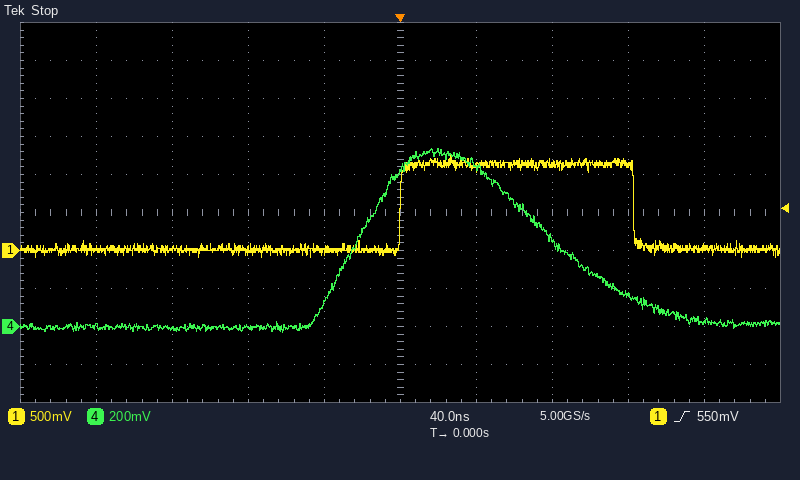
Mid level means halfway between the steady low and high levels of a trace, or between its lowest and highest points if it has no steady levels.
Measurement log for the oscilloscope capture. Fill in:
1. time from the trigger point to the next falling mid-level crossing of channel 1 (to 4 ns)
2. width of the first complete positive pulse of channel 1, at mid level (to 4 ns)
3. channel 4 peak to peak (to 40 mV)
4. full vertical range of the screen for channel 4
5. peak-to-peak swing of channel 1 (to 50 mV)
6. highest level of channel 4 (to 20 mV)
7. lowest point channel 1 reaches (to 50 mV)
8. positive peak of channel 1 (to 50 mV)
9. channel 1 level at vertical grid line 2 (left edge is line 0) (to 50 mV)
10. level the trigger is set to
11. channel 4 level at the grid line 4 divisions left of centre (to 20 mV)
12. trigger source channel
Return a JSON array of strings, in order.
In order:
["124 ns", "124 ns", "960 mV", "2 V", "1.35 V", "940 mV", "-100 mV", "1.25 V", "0 mV", "550 mV", "0 mV", "channel 1"]
